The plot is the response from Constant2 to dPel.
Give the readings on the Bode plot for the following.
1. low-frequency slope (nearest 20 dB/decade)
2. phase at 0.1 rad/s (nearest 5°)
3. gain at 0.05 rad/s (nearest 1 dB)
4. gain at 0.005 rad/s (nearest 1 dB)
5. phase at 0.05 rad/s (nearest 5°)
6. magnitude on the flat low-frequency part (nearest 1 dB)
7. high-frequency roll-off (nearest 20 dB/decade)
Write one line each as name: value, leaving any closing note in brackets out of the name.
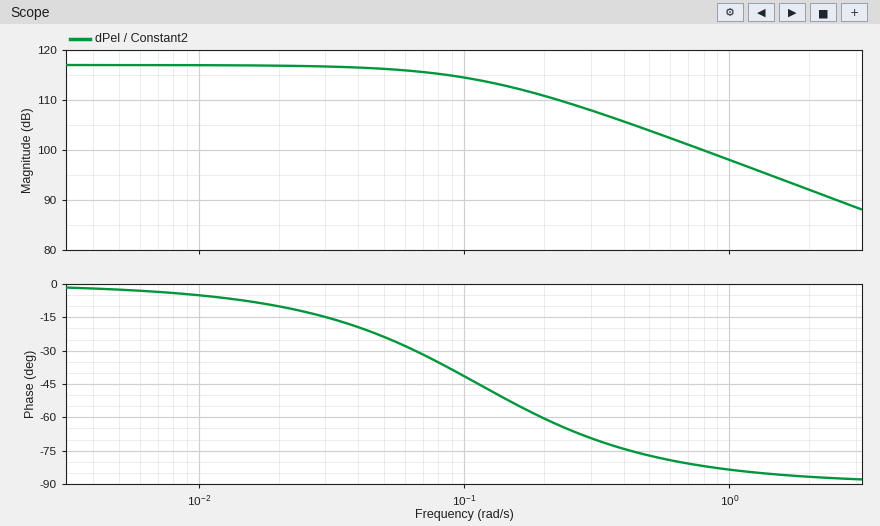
low-frequency slope: 0 dB/decade
phase at 0.1 rad/s: -40°
gain at 0.05 rad/s: 116 dB
gain at 0.005 rad/s: 117 dB
phase at 0.05 rad/s: -25°
magnitude on the flat low-frequency part: 117 dB
high-frequency roll-off: -20 dB/decade
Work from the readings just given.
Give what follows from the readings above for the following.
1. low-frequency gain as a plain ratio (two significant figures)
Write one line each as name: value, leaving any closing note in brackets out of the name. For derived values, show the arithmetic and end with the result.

low-frequency gain as a plain ratio: 10^(117 / 20) = 710000
